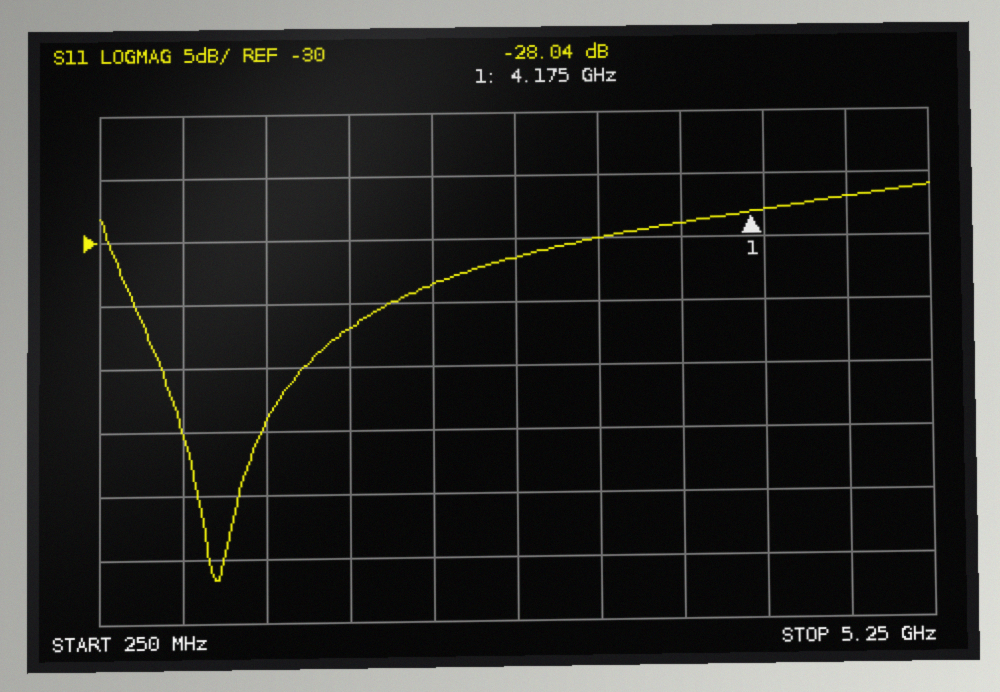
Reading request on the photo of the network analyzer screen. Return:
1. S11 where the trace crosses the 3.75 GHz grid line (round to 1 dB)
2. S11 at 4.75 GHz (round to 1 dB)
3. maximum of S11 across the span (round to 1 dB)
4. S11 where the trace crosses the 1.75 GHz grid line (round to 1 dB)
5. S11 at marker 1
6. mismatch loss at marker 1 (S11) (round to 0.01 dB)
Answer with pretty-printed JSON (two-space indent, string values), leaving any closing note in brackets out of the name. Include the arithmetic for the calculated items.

{
  "S11 where the trace crosses the 3.75 GHz grid line": "-29 dB",
  "S11 at 4.75 GHz": "-27 dB",
  "maximum of S11 across the span": "-26 dB",
  "S11 where the trace crosses the 1.75 GHz grid line": "-37 dB",
  "S11 at marker 1": "-28.04 dB",
  "mismatch loss at marker 1 (S11)": "−10 log10(1 − 10^(-28.04/10)) ≈ 0.01 dB"
}
